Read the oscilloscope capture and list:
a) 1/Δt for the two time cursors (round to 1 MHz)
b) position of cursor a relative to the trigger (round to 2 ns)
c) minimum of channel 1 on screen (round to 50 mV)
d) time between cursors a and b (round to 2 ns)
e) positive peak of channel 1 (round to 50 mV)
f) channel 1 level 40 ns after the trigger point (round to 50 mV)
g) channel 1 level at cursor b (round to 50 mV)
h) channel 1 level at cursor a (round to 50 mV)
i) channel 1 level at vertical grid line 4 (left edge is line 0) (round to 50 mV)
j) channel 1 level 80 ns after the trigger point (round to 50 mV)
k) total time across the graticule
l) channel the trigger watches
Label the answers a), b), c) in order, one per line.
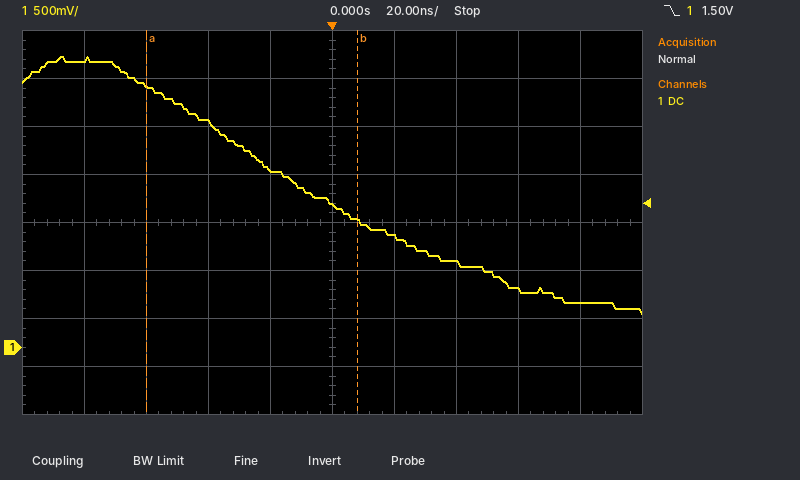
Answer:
a) 15 MHz
b) -60 ns
c) 350 mV
d) 68 ns
e) 3.05 V
f) 900 mV
g) 1.30 V
h) 2.75 V
i) 1.85 V
j) 450 mV
k) 200 ns
l) channel 1
